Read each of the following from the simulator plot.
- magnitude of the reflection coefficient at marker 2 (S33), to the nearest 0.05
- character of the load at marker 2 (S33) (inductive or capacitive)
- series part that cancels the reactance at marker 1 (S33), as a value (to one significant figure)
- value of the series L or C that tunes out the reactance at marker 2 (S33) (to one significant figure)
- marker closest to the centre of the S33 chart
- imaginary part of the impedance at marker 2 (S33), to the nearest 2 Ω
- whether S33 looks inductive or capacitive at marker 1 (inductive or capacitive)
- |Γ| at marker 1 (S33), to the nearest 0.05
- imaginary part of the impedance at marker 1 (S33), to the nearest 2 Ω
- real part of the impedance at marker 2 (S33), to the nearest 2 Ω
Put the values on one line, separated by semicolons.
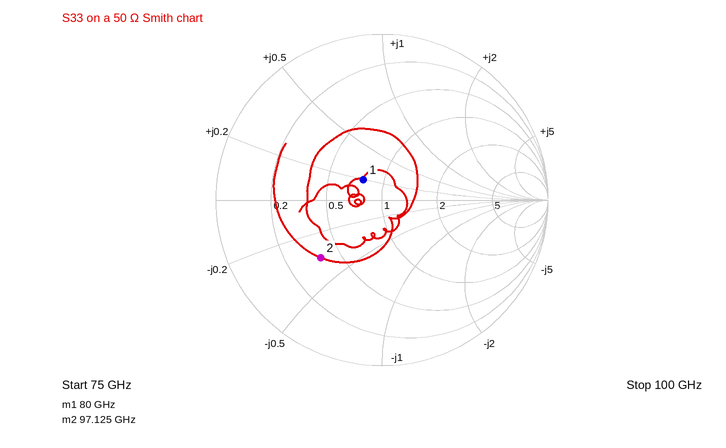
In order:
0.50; capacitive; 200 fF; 30 pH; marker 1; -18 Ω; inductive; 0.15; +10 Ω; 18 Ω
